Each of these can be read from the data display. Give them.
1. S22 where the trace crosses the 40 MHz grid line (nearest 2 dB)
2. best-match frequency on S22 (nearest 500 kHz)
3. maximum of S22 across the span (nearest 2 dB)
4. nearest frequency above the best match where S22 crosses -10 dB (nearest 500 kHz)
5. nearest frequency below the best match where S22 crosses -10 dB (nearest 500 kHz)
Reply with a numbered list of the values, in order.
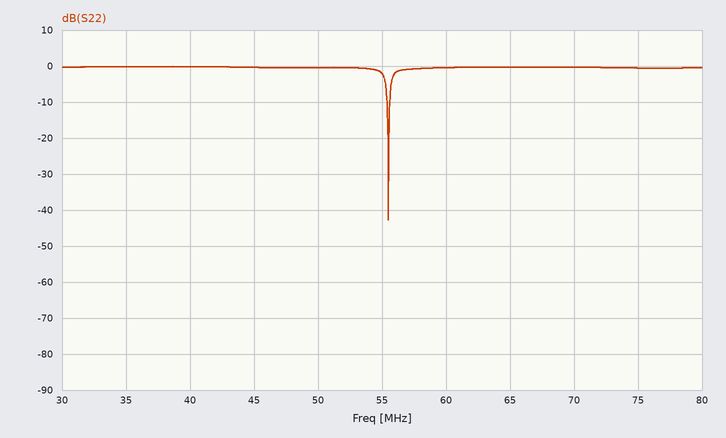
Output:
1. 0 dB
2. 55.5 MHz
3. 0 dB
4. 55.5 MHz
5. 55.5 MHz
